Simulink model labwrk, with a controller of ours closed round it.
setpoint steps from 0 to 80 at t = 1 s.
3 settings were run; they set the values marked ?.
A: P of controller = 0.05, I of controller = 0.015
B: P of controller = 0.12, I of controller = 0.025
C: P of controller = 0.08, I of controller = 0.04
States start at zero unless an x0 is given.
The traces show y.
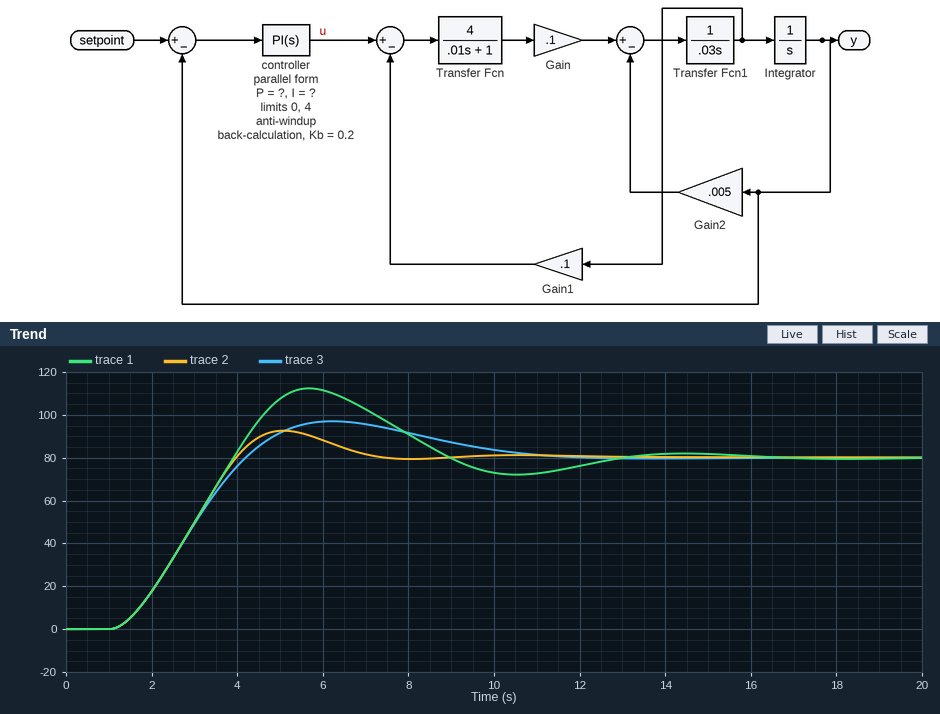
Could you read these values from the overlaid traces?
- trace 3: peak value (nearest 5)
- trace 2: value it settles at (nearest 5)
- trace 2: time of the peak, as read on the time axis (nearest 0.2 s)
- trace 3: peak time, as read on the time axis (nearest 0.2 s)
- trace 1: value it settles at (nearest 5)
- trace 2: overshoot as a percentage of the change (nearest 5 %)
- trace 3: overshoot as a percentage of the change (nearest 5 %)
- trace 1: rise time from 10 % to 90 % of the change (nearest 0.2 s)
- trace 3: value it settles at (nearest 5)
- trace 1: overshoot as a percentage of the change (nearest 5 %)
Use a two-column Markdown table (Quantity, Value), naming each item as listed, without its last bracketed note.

| Quantity | Value |
|---|---|
| trace 3: peak value | 95 |
| trace 2: value it settles at | 80 |
| trace 2: time of the peak, as read on the time axis | 5.0 s |
| trace 3: peak time, as read on the time axis | 6.2 s |
| trace 1: value it settles at | 80 |
| trace 2: overshoot as a percentage of the change | 15 % |
| trace 3: overshoot as a percentage of the change | 20 % |
| trace 1: rise time from 10 % to 90 % of the change | 2.0 s |
| trace 3: value it settles at | 80 |
| trace 1: overshoot as a percentage of the change | 40 % |
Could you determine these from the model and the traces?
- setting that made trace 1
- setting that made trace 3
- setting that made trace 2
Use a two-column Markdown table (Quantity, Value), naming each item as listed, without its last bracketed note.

| Quantity | Value |
|---|---|
| setting that made trace 1 | C |
| setting that made trace 3 | A |
| setting that made trace 2 | B |
